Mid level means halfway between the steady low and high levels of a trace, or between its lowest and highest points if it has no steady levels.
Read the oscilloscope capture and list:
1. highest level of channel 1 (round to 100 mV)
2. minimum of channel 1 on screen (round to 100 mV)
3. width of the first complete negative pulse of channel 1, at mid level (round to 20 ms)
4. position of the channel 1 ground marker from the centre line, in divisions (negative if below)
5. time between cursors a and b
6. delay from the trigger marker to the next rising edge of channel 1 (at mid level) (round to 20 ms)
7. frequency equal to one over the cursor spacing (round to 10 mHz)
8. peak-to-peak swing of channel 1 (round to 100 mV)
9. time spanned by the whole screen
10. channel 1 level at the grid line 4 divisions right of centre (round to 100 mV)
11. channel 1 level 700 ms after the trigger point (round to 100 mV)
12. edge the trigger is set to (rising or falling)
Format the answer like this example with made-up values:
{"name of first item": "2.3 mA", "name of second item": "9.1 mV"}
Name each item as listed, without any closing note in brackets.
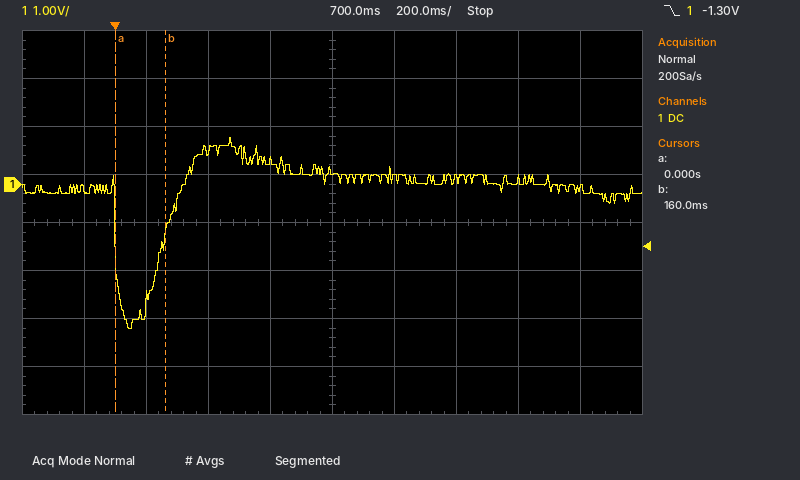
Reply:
{"highest level of channel 1": "1.0 V", "minimum of channel 1 on screen": "-3.0 V", "width of the first complete negative pulse of channel 1, at mid level": "160 ms", "position of the channel 1 ground marker from the centre line, in divisions": "+0.8 div", "time between cursors a and b": "160 ms", "delay from the trigger marker to the next rising edge of channel 1 (at mid level)": "160 ms", "frequency equal to one over the cursor spacing": "6.25 Hz", "peak-to-peak swing of channel 1": "4.0 V", "time spanned by the whole screen": "2 s", "channel 1 level at the grid line 4 divisions right of centre": "-100 mV", "channel 1 level 700 ms after the trigger point": "300 mV", "edge the trigger is set to": "falling"}
